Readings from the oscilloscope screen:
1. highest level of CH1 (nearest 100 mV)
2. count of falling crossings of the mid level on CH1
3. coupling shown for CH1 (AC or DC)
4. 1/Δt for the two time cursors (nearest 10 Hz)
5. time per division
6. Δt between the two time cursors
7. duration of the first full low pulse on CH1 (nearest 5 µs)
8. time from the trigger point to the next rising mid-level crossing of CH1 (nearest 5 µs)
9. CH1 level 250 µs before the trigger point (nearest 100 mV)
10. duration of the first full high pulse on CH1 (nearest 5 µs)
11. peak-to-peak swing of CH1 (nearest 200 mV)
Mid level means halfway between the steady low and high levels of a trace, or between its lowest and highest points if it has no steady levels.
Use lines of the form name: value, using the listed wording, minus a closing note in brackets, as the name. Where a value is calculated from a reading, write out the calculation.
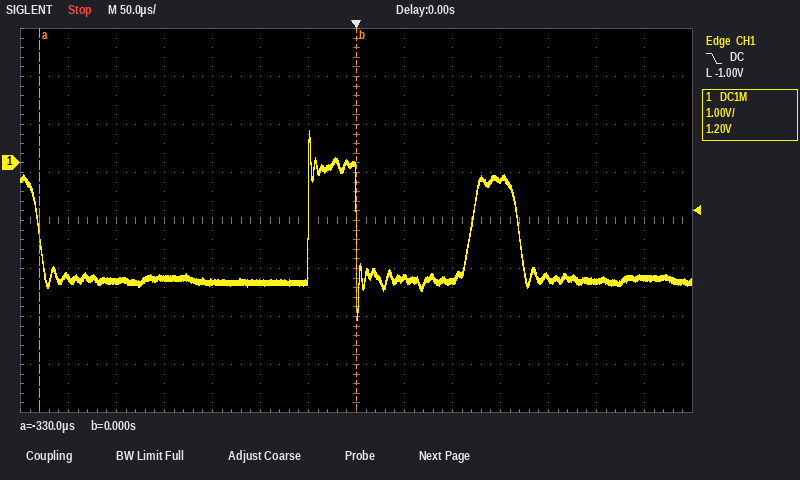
highest level of CH1: 700 mV
count of falling crossings of the mid level on CH1: 3
coupling shown for CH1: DC
1/Δt for the two time cursors: 1 / 330 µs ≈ 3.03 kHz
time per division: 50 µs
Δt between the two time cursors: 0 s − (-330 µs) = 330 µs
duration of the first full low pulse on CH1: 280 µs
time from the trigger point to the next rising mid-level crossing of CH1: 120 µs
CH1 level 250 µs before the trigger point: -2.5 V
duration of the first full high pulse on CH1: 50 µs
peak-to-peak swing of CH1: 4.0 V
